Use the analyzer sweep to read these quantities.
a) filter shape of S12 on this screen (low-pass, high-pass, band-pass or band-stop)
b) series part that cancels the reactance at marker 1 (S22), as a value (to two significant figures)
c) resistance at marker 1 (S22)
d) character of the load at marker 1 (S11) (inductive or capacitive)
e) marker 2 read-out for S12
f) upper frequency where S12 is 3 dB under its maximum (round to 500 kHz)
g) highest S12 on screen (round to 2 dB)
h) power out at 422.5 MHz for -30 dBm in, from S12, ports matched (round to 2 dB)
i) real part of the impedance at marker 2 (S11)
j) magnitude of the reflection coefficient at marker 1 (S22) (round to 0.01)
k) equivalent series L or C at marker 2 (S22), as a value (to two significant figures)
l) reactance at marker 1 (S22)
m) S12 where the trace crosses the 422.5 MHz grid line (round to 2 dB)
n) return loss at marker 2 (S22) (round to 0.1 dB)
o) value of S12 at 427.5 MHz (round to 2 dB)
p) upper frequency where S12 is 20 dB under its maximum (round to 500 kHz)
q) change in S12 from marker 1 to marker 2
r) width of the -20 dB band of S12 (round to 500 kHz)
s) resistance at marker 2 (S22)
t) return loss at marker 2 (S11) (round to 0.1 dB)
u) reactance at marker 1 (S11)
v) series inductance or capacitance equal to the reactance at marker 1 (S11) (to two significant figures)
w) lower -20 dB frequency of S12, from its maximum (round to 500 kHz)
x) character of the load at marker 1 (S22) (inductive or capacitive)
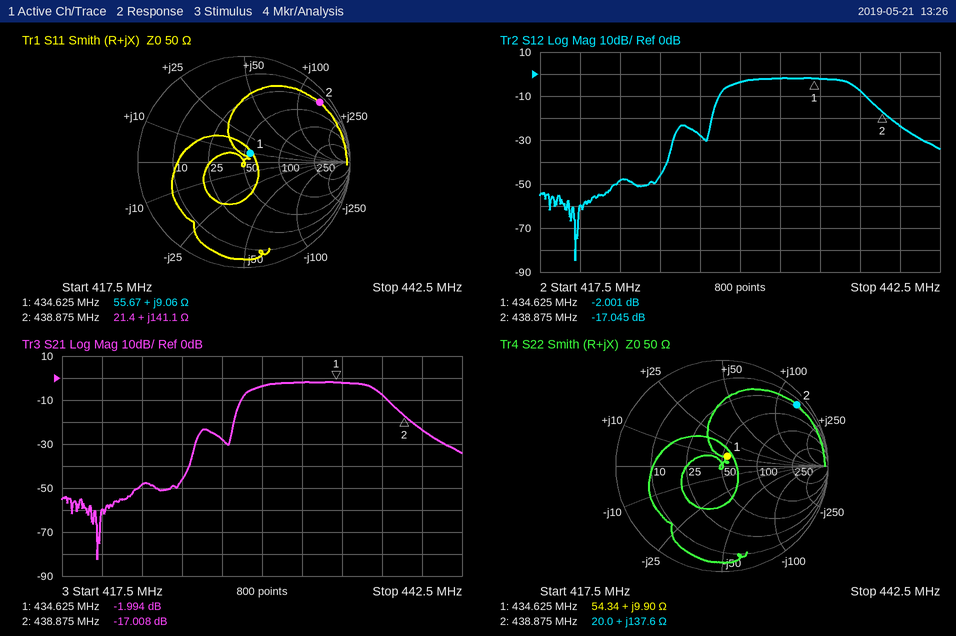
band-pass
37 pF
54.34 Ω
inductive
-17.045 dB
437.0 MHz
-2 dB
-78 dBm
21.4 Ω
0.10
50 nH
+9.90 Ω
-48 dB
0.8 dB
-28 dB
439.5 MHz
-15.044 dB
11.5 MHz
20.0 Ω
0.8 dB
+9.06 Ω
3.3 nH
428.0 MHz
inductive
